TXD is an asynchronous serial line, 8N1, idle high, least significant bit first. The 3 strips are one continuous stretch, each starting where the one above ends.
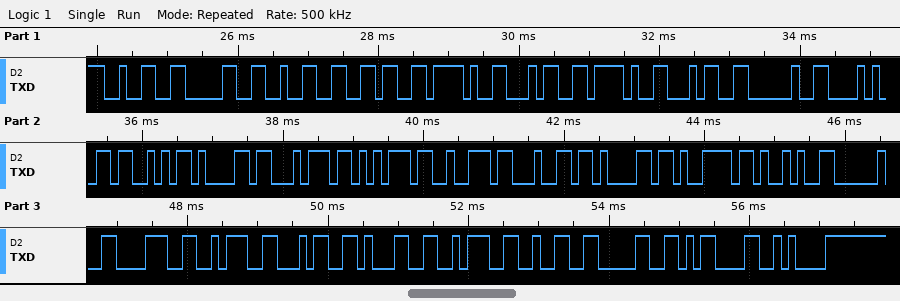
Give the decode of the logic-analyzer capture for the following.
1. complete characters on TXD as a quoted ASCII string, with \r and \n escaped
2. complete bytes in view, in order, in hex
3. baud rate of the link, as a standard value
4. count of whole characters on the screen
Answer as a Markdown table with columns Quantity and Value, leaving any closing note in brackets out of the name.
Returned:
| Quantity | Value |
|---|---|
| complete characters on TXD as a quoted ASCII string, with \r and \n escaped | "2026/4/4 (Saturday) 8:41:20\r\n" |
| complete bytes in view, in order, in hex | 32 30 32 36 2F 34 2F 34 20 28 53 61 74 75 72 64 61 79 29 20 38 3A 34 31 3A 32 30 0D 0A |
| baud rate of the link, as a standard value | 9600 baud |
| count of whole characters on the screen | 29 |
